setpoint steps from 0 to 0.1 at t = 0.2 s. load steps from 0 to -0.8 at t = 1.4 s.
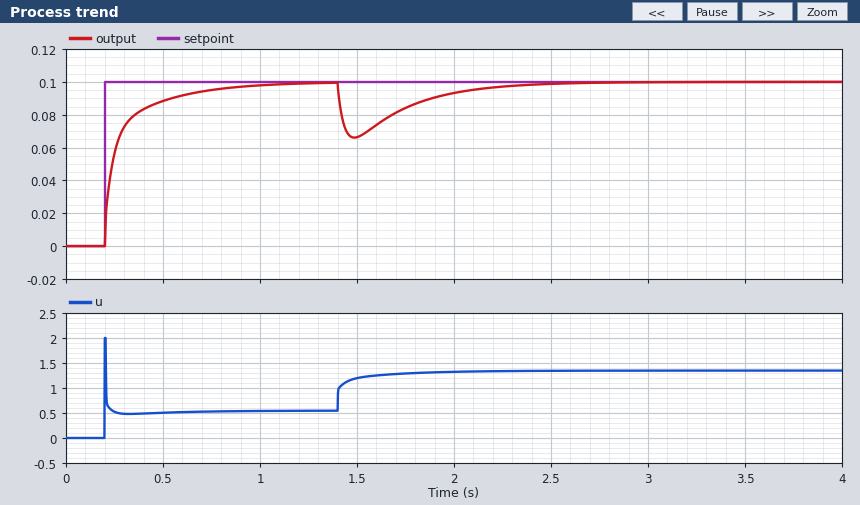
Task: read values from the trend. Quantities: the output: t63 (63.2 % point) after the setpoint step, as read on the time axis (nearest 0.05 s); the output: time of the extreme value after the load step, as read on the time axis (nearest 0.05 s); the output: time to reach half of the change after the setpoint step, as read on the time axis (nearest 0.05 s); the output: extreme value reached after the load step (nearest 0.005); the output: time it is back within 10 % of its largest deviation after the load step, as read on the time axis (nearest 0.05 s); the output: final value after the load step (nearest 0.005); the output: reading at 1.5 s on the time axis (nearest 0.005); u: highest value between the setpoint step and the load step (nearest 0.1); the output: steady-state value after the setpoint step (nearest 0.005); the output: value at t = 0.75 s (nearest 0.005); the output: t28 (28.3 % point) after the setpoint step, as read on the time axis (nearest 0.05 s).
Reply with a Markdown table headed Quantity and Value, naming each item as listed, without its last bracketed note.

| Quantity | Value |
|---|---|
| the output: t63 (63.2 % point) after the setpoint step, as read on the time axis | 0.25 s |
| the output: time of the extreme value after the load step, as read on the time axis | 1.50 s |
| the output: time to reach half of the change after the setpoint step, as read on the time axis | 0.25 s |
| the output: extreme value reached after the load step | 0.065 |
| the output: time it is back within 10 % of its largest deviation after the load step, as read on the time axis | 2.20 s |
| the output: final value after the load step | 0.100 |
| the output: reading at 1.5 s on the time axis | 0.065 |
| u: highest value between the setpoint step and the load step | 2.0 |
| the output: steady-state value after the setpoint step | 0.100 |
| the output: value at t = 0.75 s | 0.095 |
| the output: t28 (28.3 % point) after the setpoint step, as read on the time axis | 0.20 s |
